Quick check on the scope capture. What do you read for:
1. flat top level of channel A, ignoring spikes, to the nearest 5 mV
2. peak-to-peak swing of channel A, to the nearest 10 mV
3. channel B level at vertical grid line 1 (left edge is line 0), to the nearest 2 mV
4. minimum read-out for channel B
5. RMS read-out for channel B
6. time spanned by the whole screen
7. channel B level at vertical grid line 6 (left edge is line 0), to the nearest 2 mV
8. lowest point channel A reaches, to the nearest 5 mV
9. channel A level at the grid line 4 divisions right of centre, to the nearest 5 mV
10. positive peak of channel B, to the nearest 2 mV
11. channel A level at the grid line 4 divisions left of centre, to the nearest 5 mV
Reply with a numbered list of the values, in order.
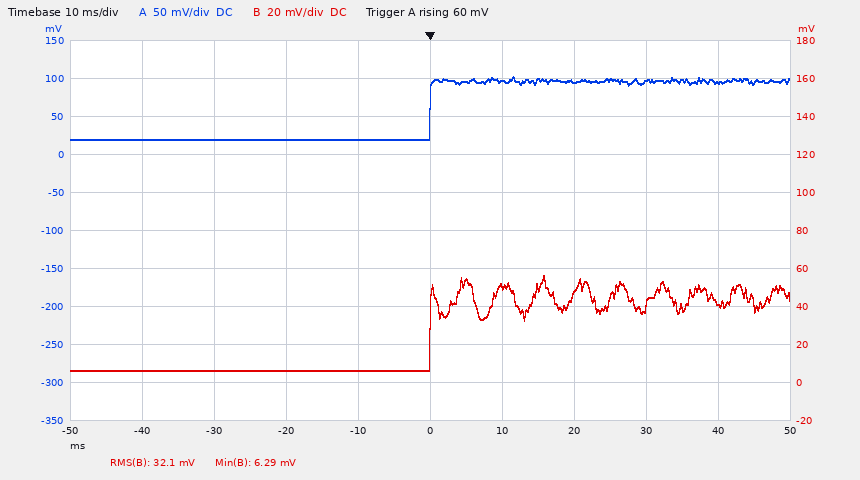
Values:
1. 95 mV
2. 80 mV
3. 6 mV
4. 6.29 mV
5. 32.1 mV
6. 100 ms
7. 50 mV
8. 20 mV
9. 95 mV
10. 56 mV
11. 20 mV
